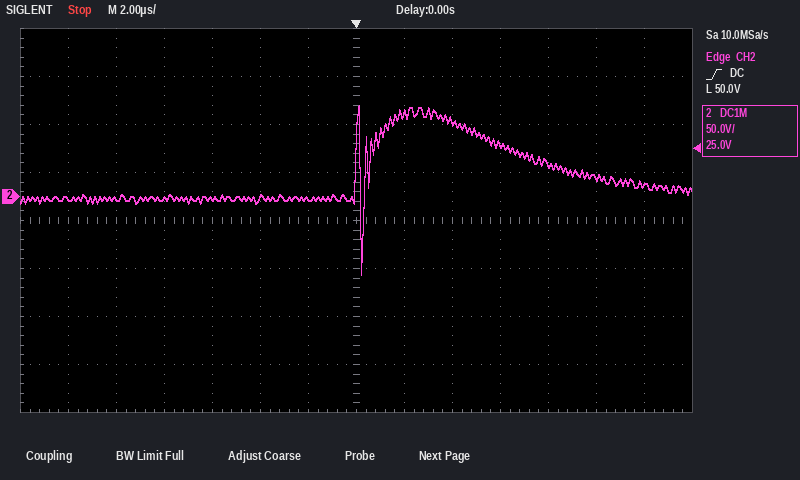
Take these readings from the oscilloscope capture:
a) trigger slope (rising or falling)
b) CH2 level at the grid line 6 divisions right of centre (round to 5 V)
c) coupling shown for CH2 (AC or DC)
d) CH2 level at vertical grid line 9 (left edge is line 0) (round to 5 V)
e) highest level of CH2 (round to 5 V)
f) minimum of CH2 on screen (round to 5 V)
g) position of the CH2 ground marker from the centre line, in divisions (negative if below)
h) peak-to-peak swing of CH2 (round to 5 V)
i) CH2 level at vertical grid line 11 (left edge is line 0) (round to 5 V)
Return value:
rising
10 V
DC
80 V
95 V
-80 V
+0.5 div
175 V
35 V
